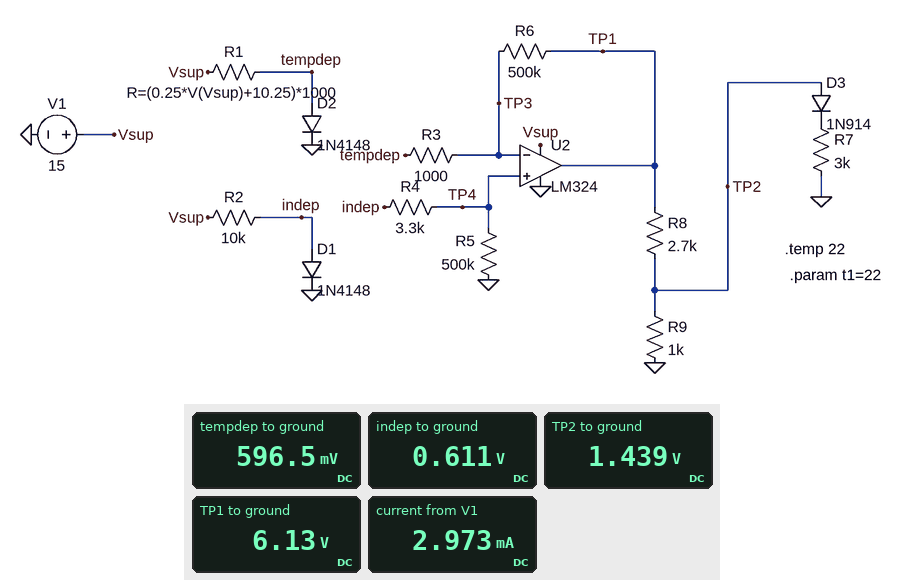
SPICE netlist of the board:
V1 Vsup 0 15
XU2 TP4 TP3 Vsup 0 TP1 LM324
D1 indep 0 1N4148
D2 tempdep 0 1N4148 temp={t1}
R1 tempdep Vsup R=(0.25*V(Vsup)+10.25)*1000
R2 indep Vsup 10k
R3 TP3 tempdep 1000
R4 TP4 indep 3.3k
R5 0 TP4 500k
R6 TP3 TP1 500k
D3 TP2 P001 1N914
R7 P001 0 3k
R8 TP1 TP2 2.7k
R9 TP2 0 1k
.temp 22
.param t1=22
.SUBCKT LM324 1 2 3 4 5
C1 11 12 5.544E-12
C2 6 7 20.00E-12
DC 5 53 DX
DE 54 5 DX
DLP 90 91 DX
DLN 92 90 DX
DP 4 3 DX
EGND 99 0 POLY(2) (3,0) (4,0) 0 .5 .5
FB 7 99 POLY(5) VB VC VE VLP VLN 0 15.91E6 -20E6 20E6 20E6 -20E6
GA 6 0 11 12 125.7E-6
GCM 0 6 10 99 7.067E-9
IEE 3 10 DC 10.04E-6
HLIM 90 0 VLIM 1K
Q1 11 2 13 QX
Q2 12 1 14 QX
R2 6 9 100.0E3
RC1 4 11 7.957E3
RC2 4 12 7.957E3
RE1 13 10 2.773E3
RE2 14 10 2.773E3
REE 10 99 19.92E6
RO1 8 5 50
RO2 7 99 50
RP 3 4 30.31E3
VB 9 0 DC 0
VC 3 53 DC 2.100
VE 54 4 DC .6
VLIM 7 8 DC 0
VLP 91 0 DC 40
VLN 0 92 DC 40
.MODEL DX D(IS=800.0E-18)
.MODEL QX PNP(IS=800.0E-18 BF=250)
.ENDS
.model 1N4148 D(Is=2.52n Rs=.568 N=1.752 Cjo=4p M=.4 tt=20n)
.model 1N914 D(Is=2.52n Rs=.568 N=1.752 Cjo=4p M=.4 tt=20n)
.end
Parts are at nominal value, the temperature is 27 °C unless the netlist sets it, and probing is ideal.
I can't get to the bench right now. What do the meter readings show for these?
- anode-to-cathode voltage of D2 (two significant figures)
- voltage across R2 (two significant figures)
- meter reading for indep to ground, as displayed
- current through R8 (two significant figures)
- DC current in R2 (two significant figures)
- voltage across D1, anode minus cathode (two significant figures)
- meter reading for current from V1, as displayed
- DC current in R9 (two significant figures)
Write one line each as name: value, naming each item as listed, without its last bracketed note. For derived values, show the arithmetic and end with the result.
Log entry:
anode-to-cathode voltage of D2: 596.5 mV = 600 mV
voltage across R2: 15 V - 611 mV = 14 V
meter reading for indep to ground, as displayed: 0.611 V
current through R8: (6.13 V - 1.439 V) / 2.7 kΩ = 1.7 mA
DC current in R2: (15 V - 611 mV) / 10 kΩ = 1.4 mA
voltage across D1, anode minus cathode: 611 mV = 610 mV
meter reading for current from V1, as displayed: 2.973 mA
DC current in R9: (1.439 V) / 1 kΩ = 1.4 mA
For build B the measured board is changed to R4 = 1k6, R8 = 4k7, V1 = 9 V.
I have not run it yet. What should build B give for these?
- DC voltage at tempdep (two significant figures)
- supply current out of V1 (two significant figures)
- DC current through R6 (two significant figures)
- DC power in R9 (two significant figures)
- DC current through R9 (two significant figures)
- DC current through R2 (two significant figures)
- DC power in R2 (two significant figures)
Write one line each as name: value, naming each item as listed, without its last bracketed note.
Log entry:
DC voltage at tempdep: 580 mV
supply current out of V1: 1.8 mA
DC current through R6: 7.7 µA
DC power in R9: 510 µW
DC current through R9: 720 µA
DC current through R2: 840 µA
DC power in R2: 7.1 mW
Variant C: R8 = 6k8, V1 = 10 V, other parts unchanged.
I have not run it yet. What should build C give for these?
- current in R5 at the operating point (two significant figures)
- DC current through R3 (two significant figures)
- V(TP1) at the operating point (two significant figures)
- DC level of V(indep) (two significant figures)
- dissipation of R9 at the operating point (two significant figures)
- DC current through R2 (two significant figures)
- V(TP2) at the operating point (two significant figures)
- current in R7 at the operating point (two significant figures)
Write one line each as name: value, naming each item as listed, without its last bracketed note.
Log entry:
current in R5 at the operating point: 1.2 µA
DC current through R3: 6.8 µA
V(TP1) at the operating point: 4.0 V
DC level of V(indep): 590 mV
dissipation of R9 at the operating point: 240 µW
DC current through R2: 940 µA
V(TP2) at the operating point: 490 mV
current in R7 at the operating point: 22 µA
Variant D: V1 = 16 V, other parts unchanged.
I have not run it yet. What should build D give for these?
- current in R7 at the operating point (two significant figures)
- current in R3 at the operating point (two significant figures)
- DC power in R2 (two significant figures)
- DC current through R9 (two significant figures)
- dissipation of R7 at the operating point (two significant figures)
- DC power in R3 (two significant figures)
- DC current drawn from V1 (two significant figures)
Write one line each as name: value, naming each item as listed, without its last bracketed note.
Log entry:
current in R7 at the operating point: 330 µA
current in R3 at the operating point: 12 µA
DC power in R2: 24 mW
DC current through R9: 1.5 mA
dissipation of R7 at the operating point: 320 µW
DC power in R3: 140 nW
DC current drawn from V1: 3.2 mA
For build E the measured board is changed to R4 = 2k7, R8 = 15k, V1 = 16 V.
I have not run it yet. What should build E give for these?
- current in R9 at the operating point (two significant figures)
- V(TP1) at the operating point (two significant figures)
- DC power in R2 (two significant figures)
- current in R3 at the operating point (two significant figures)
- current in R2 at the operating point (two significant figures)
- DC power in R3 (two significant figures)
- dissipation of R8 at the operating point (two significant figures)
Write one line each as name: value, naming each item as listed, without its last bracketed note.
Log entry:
current in R9 at the operating point: 420 µA
V(TP1) at the operating point: 6.9 V
DC power in R2: 24 mW
current in R3 at the operating point: 13 µA
current in R2 at the operating point: 1.5 mA
DC power in R3: 160 nW
dissipation of R8 at the operating point: 2.8 mW
